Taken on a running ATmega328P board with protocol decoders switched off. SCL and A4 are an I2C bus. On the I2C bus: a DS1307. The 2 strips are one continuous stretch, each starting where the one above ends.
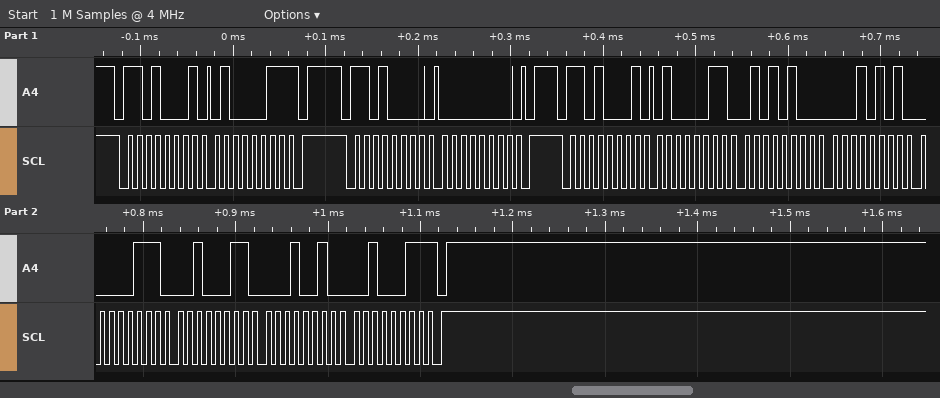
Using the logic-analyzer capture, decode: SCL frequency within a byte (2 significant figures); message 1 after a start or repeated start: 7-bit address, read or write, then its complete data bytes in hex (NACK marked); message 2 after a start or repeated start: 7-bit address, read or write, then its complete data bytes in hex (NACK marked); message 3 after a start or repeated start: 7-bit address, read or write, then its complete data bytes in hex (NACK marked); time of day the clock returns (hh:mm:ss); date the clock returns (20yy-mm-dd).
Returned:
100 kHz
0x68 read: 43 NACK
0x68 write: 00
0x68 read: 43 54 15 07 23 12 23 NACK
15:54:43
2023-12-23
